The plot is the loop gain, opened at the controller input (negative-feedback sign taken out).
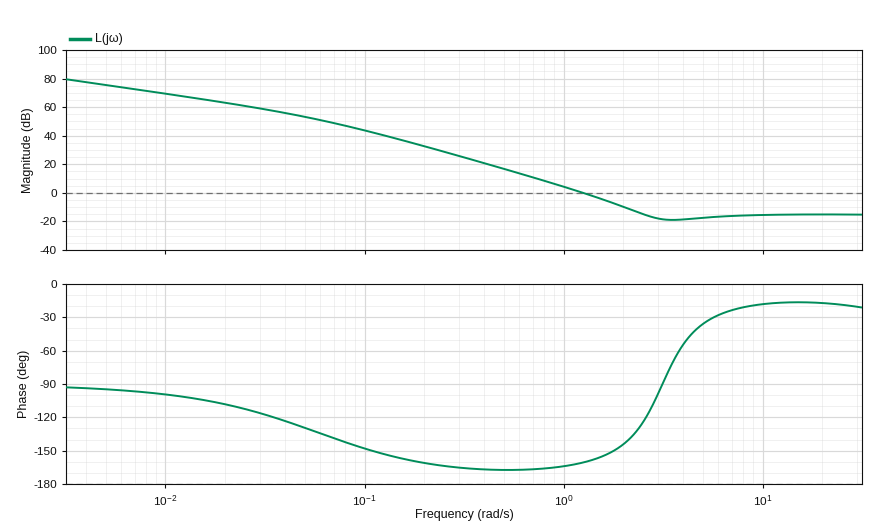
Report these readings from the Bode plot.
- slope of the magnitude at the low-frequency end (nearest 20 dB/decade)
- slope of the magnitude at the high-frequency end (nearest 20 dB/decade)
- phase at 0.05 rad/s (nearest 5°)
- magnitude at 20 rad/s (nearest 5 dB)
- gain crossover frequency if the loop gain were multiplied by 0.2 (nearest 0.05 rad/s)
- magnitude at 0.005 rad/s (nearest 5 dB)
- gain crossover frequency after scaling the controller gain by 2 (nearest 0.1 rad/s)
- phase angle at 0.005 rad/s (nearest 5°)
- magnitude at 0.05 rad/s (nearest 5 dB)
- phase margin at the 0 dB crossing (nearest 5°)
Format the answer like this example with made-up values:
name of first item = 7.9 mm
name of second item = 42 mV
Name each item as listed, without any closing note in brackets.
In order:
slope of the magnitude at the low-frequency end = -20 dB/decade
slope of the magnitude at the high-frequency end = 0 dB/decade
phase at 0.05 rad/s = -130°
magnitude at 20 rad/s = -15 dB
gain crossover frequency if the loop gain were multiplied by 0.2 = 0.60 rad/s
magnitude at 0.005 rad/s = 75 dB
gain crossover frequency after scaling the controller gain by 2 = 1.7 rad/s
phase angle at 0.005 rad/s = -95°
magnitude at 0.05 rad/s = 55 dB
phase margin at the 0 dB crossing = 20°
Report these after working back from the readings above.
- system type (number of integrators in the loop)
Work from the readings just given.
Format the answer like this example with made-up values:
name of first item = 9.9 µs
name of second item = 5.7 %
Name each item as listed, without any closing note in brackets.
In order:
system type = 1
